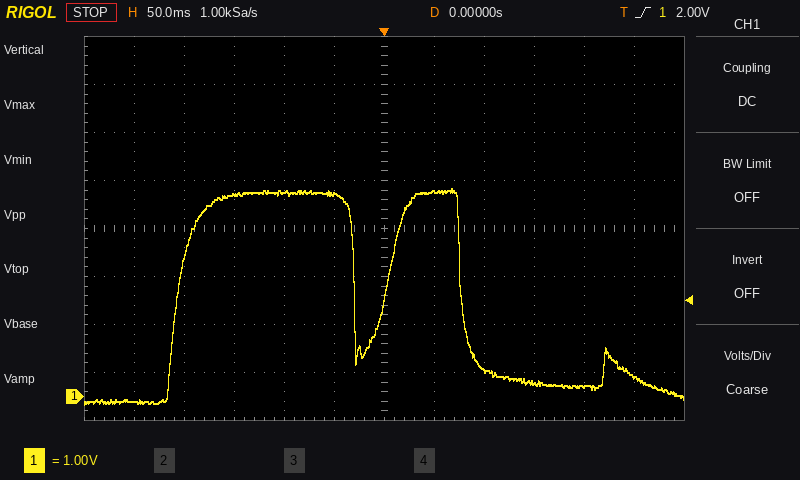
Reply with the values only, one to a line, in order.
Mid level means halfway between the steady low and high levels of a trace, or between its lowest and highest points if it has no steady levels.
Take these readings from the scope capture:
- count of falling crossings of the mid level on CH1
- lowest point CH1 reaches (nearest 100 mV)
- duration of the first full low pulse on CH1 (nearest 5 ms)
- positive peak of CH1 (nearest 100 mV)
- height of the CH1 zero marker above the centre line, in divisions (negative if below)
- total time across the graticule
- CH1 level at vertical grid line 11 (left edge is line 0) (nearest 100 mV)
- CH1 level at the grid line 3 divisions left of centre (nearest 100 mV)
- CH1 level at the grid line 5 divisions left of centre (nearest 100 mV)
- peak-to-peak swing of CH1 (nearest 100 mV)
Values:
2
-200 mV
30 ms
4.3 V
-3.5 div
600 ms
400 mV
4.2 V
-100 mV
4.5 V
